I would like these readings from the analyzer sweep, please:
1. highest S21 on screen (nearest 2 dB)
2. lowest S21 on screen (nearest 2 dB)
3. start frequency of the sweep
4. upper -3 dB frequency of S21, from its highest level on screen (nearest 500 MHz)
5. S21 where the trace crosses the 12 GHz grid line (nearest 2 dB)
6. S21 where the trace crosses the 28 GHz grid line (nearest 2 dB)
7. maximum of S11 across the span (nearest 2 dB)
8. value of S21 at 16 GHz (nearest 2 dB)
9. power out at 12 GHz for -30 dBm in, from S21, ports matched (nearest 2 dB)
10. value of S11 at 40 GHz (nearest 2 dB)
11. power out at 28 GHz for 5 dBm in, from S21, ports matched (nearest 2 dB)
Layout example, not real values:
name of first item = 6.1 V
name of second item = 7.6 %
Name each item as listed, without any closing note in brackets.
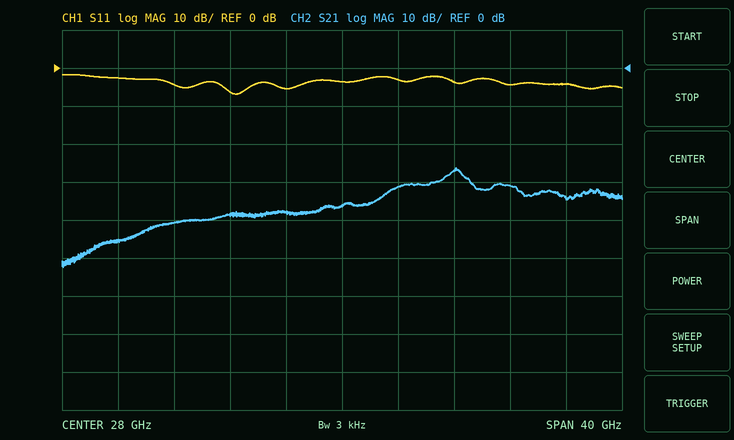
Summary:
highest S21 on screen = -26 dB
lowest S21 on screen = -52 dB
start frequency of the sweep = 8 GHz
upper -3 dB frequency of S21, from its highest level on screen = 37.0 GHz
S21 where the trace crosses the 12 GHz grid line = -46 dB
S21 where the trace crosses the 28 GHz grid line = -36 dB
maximum of S11 across the span = -2 dB
value of S21 at 16 GHz = -40 dB
power out at 12 GHz for -30 dBm in, from S21, ports matched = -76 dBm
value of S11 at 40 GHz = -4 dB
power out at 28 GHz for 5 dBm in, from S21, ports matched = -32 dBm
